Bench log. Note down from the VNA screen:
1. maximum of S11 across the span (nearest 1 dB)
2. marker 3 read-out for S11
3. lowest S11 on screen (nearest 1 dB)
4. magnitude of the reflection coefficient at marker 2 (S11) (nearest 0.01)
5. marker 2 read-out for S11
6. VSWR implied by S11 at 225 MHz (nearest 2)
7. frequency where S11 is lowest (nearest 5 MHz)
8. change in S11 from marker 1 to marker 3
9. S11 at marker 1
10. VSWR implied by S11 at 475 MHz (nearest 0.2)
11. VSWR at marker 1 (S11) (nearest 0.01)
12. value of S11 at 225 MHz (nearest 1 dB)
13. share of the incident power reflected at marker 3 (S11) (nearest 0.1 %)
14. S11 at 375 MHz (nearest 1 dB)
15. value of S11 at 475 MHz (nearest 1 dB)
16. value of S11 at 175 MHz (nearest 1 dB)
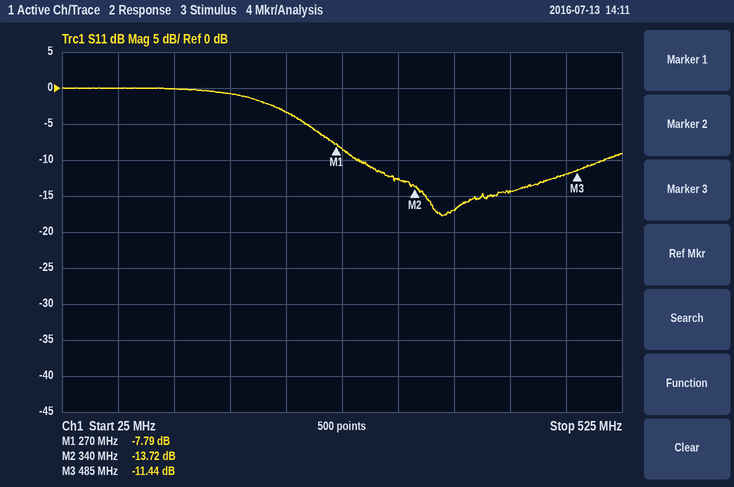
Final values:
0 dB
-11.44 dB
-18 dB
0.21
-13.72 dB
6
365 MHz
-3.65 dB
-7.79 dB
1.6
2.38
-3 dB
7.2 %
-17 dB
-12 dB
-1 dB
